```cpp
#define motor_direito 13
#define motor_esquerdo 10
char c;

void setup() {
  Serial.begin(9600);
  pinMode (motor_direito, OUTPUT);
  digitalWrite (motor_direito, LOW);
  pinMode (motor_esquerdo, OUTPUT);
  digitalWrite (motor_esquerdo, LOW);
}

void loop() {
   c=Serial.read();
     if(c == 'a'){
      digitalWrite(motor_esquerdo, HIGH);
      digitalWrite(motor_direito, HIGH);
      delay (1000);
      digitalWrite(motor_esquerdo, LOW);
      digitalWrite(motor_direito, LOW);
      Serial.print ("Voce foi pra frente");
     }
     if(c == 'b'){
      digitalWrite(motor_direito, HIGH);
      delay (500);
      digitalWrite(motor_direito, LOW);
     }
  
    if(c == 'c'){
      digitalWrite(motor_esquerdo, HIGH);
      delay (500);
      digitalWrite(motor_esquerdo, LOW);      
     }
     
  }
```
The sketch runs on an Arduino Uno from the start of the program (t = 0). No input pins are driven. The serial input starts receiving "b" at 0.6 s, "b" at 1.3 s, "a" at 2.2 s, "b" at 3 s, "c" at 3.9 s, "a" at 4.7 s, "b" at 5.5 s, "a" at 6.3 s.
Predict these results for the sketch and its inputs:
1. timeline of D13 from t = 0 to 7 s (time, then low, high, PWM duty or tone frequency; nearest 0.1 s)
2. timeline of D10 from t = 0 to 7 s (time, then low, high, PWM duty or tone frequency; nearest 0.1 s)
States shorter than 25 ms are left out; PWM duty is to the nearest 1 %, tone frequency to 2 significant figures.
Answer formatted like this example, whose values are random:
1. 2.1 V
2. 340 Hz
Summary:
1. 0 s low; 0.6 s high; 1.1 s low; 1.3 s high; 1.8 s low; 2.2 s high; 3.7 s low; 4.7 s high; 6.2 s low; 6.3 s high
2. 0 s low; 2.2 s high; 3.2 s low; 3.9 s high; 4.4 s low; 4.7 s high; 5.7 s low; 6.3 s high
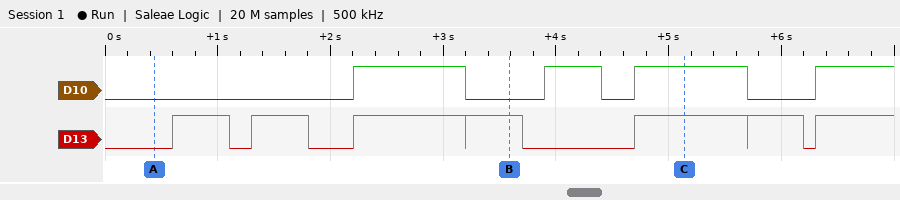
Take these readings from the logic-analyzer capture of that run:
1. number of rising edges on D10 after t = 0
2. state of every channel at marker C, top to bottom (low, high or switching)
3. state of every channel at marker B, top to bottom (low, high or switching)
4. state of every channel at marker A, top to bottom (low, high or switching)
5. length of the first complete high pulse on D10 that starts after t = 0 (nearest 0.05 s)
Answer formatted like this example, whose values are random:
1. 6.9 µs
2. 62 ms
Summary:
1. 4
2. D10 high, D13 high
3. D10 low, D13 high
4. D10 low, D13 low
5. 1.00 s
